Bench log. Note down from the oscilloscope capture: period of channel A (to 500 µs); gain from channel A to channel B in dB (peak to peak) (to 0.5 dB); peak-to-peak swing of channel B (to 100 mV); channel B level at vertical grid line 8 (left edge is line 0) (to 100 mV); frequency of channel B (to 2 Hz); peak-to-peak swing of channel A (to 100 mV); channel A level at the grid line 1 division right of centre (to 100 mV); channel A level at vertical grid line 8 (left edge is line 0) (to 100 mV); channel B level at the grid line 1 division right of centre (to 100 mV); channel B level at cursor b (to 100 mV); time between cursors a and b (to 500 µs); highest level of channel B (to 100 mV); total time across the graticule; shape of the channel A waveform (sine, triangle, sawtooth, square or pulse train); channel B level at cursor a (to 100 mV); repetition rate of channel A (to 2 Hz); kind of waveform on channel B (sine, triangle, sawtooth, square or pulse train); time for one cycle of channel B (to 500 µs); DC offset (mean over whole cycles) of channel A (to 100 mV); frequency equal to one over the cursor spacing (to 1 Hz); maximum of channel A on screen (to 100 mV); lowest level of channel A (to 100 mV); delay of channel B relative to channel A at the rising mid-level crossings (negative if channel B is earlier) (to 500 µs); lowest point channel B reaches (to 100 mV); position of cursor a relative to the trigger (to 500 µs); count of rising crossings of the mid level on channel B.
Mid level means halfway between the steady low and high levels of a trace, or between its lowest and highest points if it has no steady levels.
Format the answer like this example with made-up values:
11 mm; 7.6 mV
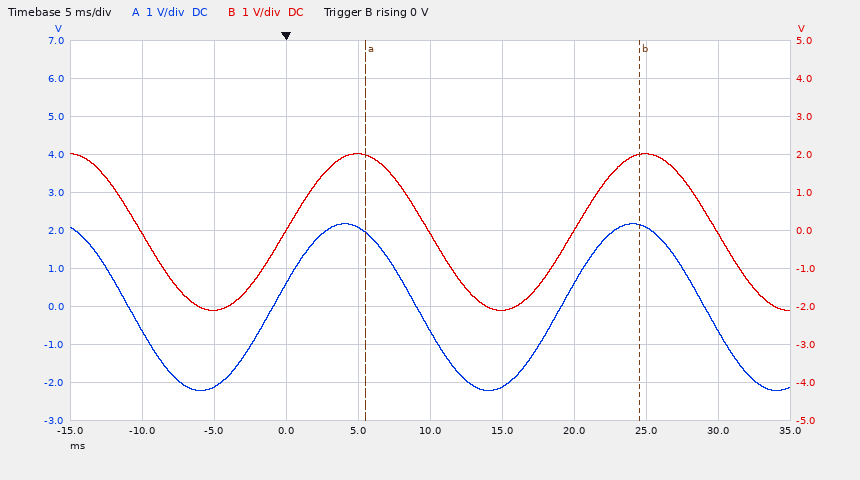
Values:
20.0 ms; -0.5 dB; 4.1 V; 2.0 V; 50 Hz; 4.4 V; -2.1 V; 2.1 V; -2.1 V; 2.0 V; 19.0 ms; 2.0 V; 50 ms; sine; 2.0 V; 50 Hz; sine; 20.0 ms; 0.0 V; 53 Hz; 2.2 V; -2.2 V; +1.0 ms; -2.1 V; +5.5 ms; 2
